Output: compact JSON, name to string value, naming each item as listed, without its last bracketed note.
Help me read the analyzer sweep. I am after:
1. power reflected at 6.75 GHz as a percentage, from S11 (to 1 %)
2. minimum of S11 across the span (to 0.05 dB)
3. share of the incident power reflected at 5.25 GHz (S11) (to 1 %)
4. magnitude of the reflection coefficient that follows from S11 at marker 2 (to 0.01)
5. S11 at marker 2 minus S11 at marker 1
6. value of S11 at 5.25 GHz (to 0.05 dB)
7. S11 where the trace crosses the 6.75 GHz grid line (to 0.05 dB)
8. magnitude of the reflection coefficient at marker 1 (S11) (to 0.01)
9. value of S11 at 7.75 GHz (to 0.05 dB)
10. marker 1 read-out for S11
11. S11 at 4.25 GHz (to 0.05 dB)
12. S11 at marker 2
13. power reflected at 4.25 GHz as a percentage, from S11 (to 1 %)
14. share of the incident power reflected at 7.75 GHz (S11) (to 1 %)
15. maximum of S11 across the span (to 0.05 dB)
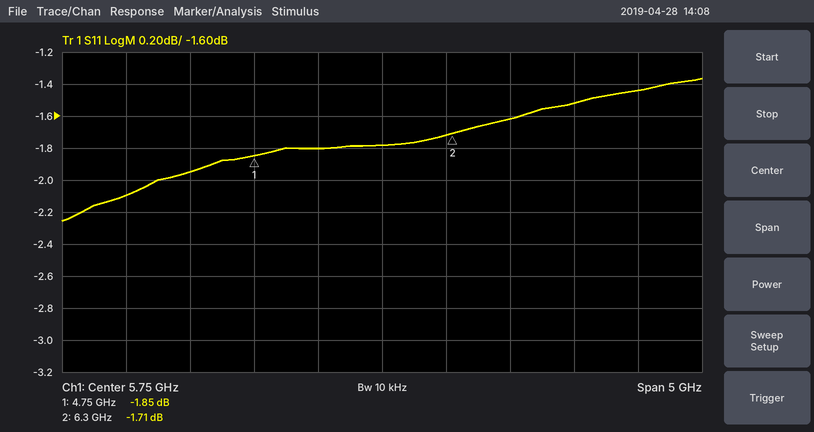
{"power reflected at 6.75 GHz as a percentage, from S11": "69 %", "minimum of S11 across the span": "-2.25 dB", "share of the incident power reflected at 5.25 GHz (S11)": "66 %", "magnitude of the reflection coefficient that follows from S11 at marker 2": "0.82", "S11 at marker 2 minus S11 at marker 1": "0.14 dB", "value of S11 at 5.25 GHz": "-1.80 dB", "S11 where the trace crosses the 6.75 GHz grid line": "-1.60 dB", "magnitude of the reflection coefficient at marker 1 (S11)": "0.81", "value of S11 at 7.75 GHz": "-1.45 dB", "marker 1 read-out for S11": "-1.85 dB", "S11 at 4.25 GHz": "-1.95 dB", "S11 at marker 2": "-1.71 dB", "power reflected at 4.25 GHz as a percentage, from S11": "64 %", "share of the incident power reflected at 7.75 GHz (S11)": "72 %", "maximum of S11 across the span": "-1.35 dB"}
